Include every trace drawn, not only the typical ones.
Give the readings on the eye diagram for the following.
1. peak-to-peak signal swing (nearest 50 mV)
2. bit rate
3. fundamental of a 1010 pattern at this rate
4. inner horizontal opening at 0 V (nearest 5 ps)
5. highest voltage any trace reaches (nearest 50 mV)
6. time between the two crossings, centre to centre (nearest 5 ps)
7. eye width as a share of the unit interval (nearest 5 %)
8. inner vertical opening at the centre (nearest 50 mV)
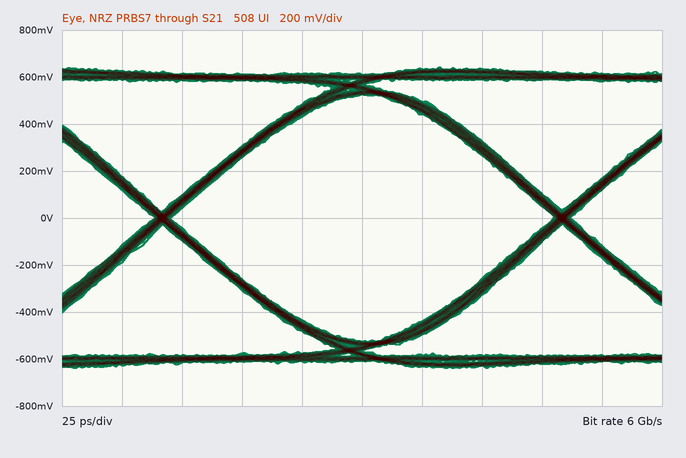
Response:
1.30 V
6 Gb/s
3 GHz
160 ps
650 mV
165 ps
95 %
1.05 V
